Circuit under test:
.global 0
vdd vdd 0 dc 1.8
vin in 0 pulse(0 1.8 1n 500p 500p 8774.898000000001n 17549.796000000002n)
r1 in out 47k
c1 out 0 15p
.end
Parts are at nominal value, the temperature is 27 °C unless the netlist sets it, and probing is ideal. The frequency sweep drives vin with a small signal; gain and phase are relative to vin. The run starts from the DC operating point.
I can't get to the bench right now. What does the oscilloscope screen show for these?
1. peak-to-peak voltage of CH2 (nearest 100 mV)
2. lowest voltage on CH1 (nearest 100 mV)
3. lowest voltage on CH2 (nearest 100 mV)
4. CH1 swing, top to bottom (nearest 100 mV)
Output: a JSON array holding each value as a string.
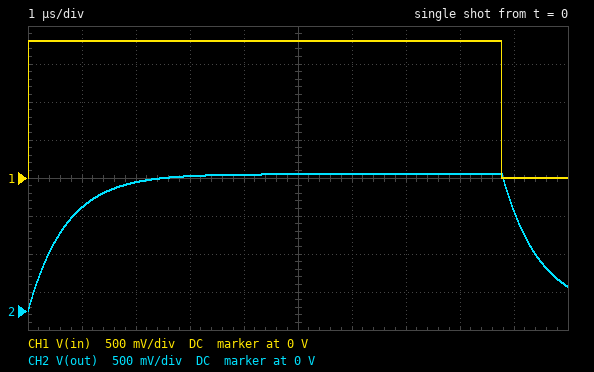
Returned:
["1.8 V", "0 V", "0 V", "1.8 V"]
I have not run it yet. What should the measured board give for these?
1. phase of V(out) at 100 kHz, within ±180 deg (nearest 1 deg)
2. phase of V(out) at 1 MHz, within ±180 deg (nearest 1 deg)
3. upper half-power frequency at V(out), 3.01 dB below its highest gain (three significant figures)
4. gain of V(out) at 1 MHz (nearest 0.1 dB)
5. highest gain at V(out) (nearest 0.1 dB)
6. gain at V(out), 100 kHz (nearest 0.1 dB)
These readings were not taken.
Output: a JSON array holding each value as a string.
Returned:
["-24 deg", "-77 deg", "226 kHz", "-13.1 dB", "0 dB", "-0.8 dB"]
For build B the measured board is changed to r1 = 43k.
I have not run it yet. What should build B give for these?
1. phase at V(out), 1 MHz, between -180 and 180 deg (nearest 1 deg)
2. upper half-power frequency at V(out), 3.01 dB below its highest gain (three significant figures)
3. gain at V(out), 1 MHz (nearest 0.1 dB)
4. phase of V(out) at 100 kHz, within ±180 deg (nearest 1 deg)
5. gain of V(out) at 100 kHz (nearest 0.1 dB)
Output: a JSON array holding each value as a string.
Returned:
["-76 deg", "247 kHz", "-12.4 dB", "-22 deg", "-0.7 dB"]
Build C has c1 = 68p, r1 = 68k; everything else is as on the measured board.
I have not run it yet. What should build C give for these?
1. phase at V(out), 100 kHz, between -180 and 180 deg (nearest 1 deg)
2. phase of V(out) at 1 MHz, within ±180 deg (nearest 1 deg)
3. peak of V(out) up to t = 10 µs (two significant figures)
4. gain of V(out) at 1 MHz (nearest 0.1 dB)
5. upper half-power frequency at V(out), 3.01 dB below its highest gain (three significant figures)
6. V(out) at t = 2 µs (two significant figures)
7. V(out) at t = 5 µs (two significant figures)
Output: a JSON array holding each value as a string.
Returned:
["-71 deg", "-88 deg", "1.5 V", "-29.3 dB", "34.4 kHz", "630 mV", "1.2 V"]
